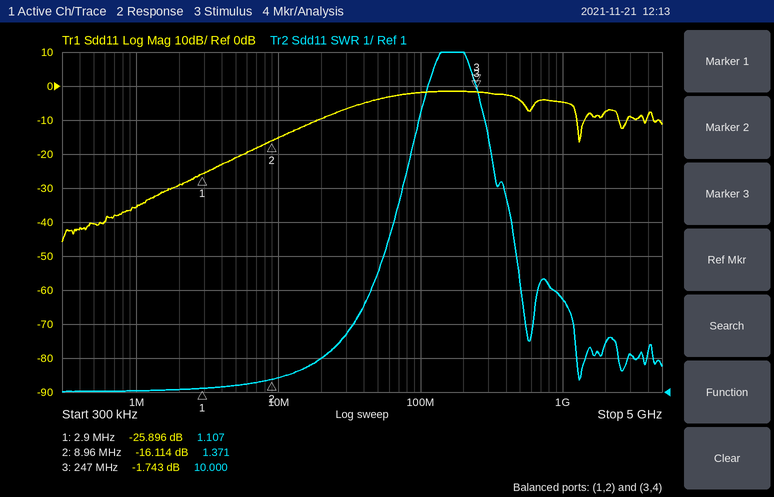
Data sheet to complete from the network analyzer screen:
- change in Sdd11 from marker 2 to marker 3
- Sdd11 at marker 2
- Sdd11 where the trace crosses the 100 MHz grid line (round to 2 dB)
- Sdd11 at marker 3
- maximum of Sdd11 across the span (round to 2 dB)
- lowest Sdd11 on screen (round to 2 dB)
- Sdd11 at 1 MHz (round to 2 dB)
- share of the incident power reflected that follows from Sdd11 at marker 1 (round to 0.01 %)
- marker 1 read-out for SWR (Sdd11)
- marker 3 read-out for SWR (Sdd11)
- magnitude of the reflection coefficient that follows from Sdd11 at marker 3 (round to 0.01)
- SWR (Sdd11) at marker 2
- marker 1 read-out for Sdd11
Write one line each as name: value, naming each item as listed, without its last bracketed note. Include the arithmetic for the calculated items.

change in Sdd11 from marker 2 to marker 3: -1.743 − (-16.114) = 14.371 dB
Sdd11 at marker 2: -16.114 dB
Sdd11 where the trace crosses the 100 MHz grid line: -2 dB
Sdd11 at marker 3: -1.743 dB
maximum of Sdd11 across the span: -2 dB
lowest Sdd11 on screen: -46 dB
Sdd11 at 1 MHz: -36 dB
share of the incident power reflected that follows from Sdd11 at marker 1: 10^(-25.896/10) ≈ 0.26 %
marker 1 read-out for SWR: 1.107
marker 3 read-out for SWR: 10.000
magnitude of the reflection coefficient that follows from Sdd11 at marker 3: 10^(-1.743/20) ≈ 0.82
SWR (Sdd11) at marker 2: 1.371
marker 1 read-out for Sdd11: -25.896 dB
